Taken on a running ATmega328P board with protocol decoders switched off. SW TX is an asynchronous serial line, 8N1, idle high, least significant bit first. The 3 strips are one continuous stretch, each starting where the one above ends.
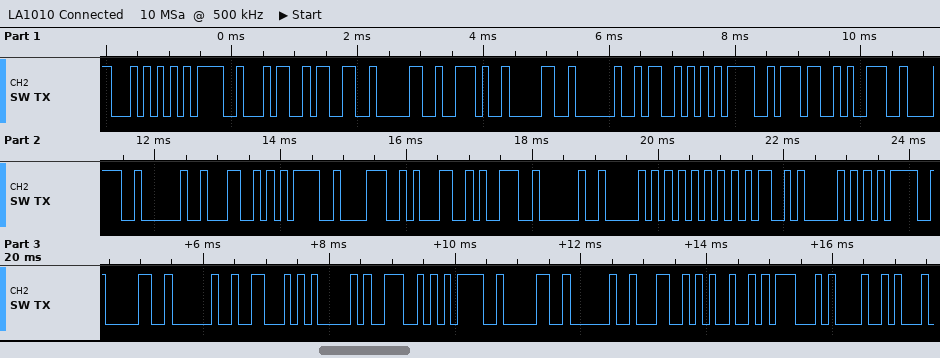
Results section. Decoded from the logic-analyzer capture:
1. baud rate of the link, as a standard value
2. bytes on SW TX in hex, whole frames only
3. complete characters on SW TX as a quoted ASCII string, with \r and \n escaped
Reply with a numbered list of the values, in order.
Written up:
1. 9600 baud
2. 0x54 0x3D 0x34 0x33 0x30 0x2E 0x30 0x20 0x53 0x3D 0x37 0x39 0x38 0x20 0x4C 0x3D 0x38 0x31 0x39 0x20 0x50 0x55 0x4D 0x50 0x3D 0x30 0x20 0x46 0x41 0x4E 0x3D 0x30 0x20 0x4C 0x49 0x47 0x48
3. "T=430.0 S=798 L=819 PUMP=0 FAN=0 LIGH"
